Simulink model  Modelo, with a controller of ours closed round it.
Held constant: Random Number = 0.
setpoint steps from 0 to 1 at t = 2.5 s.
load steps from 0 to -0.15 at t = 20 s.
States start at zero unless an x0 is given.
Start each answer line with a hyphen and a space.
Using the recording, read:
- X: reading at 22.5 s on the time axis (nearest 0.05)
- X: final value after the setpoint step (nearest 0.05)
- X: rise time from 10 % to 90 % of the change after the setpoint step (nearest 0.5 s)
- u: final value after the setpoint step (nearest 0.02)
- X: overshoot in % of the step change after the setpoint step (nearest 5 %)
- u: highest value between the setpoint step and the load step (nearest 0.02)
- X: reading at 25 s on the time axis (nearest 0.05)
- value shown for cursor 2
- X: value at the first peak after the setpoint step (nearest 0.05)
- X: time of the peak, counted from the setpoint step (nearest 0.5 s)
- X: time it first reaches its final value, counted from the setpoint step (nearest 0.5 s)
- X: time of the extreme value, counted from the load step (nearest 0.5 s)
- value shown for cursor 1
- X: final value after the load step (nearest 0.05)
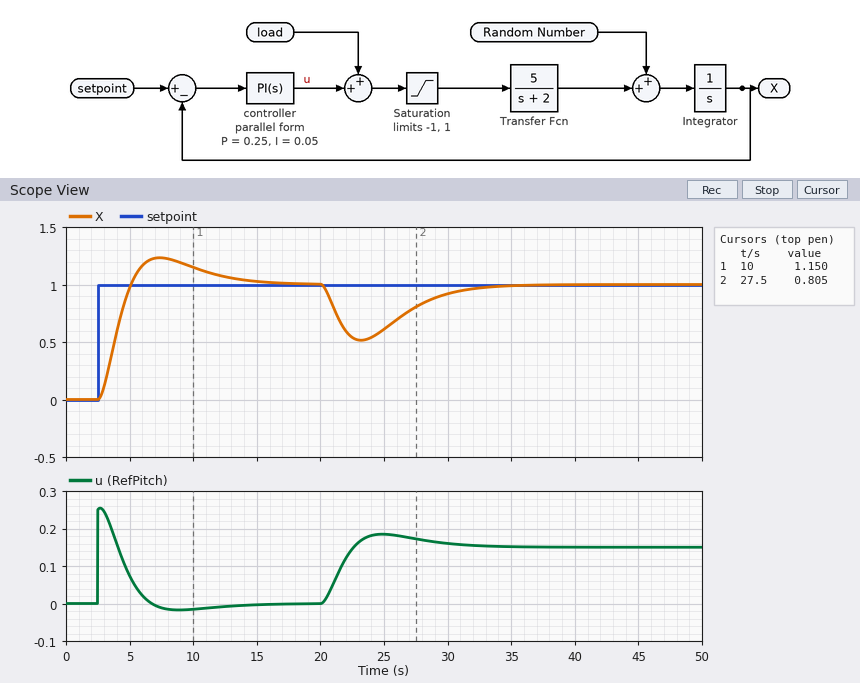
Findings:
- 0.55
- 1.00
- 2.0 s
- 0.00
- 25 %
- 0.26
- 0.60
- 0.805
- 1.25
- 5.0 s
- 2.5 s
- 3.0 s
- 1.150
- 1.00
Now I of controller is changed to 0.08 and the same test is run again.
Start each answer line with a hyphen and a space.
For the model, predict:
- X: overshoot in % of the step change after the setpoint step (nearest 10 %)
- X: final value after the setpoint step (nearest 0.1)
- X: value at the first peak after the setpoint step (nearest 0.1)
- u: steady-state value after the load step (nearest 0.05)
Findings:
- 30 %
- 1.0
- 1.3
- 0.15
